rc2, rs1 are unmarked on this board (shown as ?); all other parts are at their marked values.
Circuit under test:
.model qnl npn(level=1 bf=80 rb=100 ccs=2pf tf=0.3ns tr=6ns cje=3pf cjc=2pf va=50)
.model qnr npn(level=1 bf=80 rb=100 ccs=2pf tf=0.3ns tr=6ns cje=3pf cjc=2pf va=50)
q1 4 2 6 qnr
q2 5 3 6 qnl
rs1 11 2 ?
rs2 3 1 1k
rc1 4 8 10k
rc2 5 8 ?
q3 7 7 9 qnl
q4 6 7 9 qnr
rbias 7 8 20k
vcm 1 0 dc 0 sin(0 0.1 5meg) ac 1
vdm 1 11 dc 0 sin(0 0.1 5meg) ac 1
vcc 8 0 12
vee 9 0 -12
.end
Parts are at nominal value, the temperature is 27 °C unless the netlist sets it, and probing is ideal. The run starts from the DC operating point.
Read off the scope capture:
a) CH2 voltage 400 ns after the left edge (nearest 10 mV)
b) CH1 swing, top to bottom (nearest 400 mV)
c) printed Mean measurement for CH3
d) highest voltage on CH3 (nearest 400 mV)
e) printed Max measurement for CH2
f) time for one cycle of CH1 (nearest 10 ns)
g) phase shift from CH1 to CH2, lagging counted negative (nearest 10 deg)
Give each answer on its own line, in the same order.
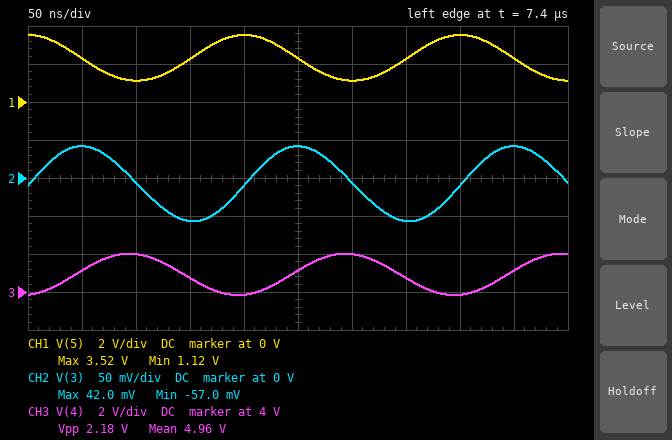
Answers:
-10 mV
2.4 V
4.96 V
6.0 V
42.0 mV
200 ns
-90 deg
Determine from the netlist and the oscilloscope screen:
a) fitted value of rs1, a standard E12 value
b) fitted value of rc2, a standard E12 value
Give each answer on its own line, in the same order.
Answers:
820 Ω
15 kΩ
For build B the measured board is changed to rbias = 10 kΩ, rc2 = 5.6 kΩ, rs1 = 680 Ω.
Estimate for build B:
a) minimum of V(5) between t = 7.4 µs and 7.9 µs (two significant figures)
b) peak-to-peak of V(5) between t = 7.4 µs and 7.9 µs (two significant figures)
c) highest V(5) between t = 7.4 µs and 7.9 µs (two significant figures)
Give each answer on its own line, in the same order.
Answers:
2.8 V
1.8 V
4.6 V
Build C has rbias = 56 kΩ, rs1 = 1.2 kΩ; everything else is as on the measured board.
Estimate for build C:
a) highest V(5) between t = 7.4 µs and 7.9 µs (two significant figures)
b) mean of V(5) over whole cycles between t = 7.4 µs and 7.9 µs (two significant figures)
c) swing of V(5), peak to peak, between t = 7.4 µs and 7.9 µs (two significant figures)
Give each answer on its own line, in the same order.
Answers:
9.5 V
8.4 V
2.3 V
